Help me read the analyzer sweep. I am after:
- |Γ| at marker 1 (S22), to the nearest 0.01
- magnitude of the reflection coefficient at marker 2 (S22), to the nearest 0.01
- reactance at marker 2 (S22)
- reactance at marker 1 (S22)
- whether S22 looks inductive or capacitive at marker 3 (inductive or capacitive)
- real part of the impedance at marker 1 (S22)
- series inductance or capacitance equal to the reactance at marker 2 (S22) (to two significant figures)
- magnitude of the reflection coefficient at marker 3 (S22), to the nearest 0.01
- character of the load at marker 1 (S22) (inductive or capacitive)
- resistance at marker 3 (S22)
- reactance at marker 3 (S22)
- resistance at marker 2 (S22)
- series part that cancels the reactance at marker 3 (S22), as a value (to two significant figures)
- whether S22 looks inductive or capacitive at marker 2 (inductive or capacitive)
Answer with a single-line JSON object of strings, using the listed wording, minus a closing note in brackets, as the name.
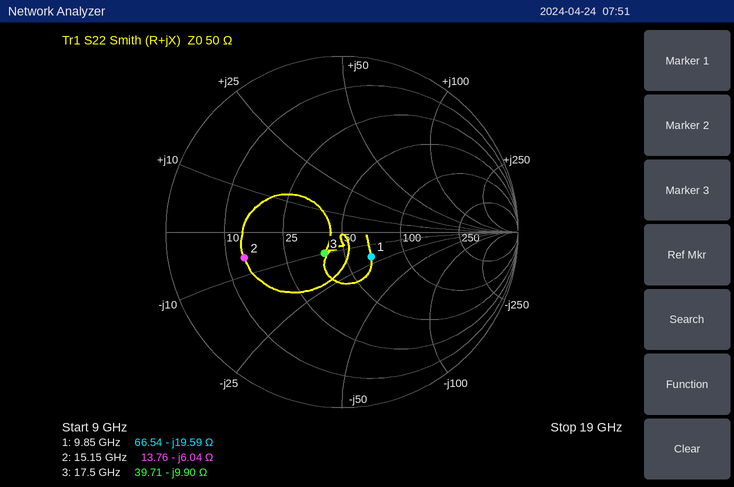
{"|Γ| at marker 1 (S22), to the nearest 0.01": "0.22", "magnitude of the reflection coefficient at marker 2 (S22), to the nearest 0.01": "0.57", "reactance at marker 2": "-6.04 Ω", "reactance at marker 1": "-19.59 Ω", "whether S22 looks inductive or capacitive at marker 3": "capacitive", "real part of the impedance at marker 1": "66.54 Ω", "series inductance or capacitance equal to the reactance at marker 2 (S22)": "1.7 pF", "magnitude of the reflection coefficient at marker 3 (S22), to the nearest 0.01": "0.16", "character of the load at marker 1 (S22)": "capacitive", "resistance at marker 3": "39.71 Ω", "reactance at marker 3": "-9.90 Ω", "resistance at marker 2": "13.76 Ω", "series part that cancels the reactance at marker 3 (S22), as a value": "90 pH", "whether S22 looks inductive or capacitive at marker 2": "capacitive"}
